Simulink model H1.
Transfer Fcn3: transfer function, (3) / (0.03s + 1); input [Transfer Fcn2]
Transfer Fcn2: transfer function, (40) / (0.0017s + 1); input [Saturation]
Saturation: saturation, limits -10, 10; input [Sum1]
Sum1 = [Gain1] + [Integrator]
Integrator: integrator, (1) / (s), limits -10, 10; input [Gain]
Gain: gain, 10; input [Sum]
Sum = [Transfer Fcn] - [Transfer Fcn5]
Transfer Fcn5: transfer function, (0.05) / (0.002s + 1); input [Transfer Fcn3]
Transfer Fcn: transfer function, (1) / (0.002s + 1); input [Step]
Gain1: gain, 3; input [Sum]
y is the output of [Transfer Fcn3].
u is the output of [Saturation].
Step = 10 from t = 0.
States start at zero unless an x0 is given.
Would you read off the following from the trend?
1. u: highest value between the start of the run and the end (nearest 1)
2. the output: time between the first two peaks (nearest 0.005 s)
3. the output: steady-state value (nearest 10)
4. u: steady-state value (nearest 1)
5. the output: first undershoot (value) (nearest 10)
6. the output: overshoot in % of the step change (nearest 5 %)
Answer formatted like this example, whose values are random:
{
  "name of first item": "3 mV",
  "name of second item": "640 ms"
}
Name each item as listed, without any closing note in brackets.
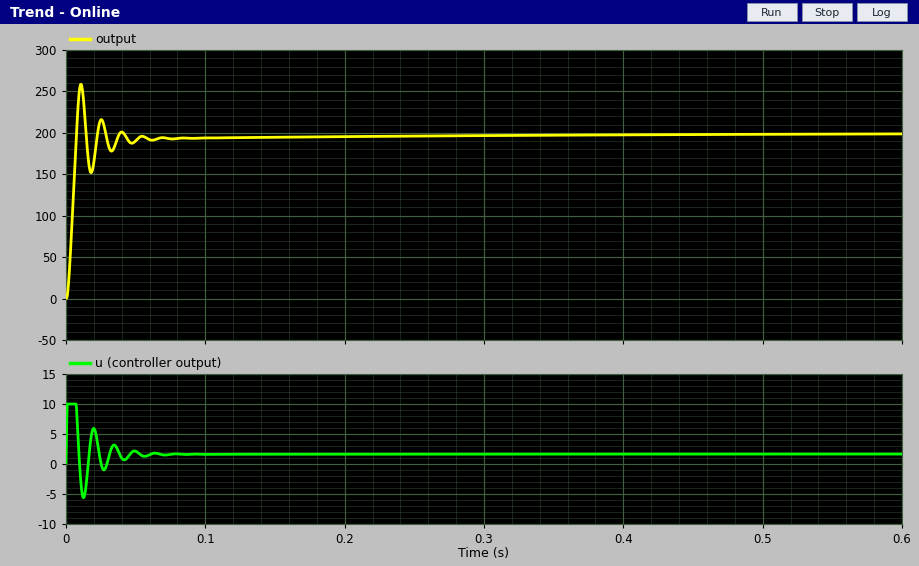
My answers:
{
  "u: highest value between the start of the run and the end": "10",
  "the output: time between the first two peaks": "0.015 s",
  "the output: steady-state value": "200",
  "u: steady-state value": "2",
  "the output: first undershoot (value)": "150",
  "the output: overshoot in % of the step change": "30 %"
}
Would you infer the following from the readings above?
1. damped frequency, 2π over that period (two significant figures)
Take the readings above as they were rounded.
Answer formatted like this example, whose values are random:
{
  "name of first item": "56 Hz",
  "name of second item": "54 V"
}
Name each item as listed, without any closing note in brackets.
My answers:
{
  "damped frequency, 2π over that period": "420 rad/s"
}
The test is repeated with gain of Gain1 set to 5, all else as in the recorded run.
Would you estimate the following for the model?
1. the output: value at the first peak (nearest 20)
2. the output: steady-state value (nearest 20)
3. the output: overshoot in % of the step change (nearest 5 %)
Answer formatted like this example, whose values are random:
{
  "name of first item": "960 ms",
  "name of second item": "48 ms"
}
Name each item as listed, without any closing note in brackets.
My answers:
{
  "the output: value at the first peak": "260",
  "the output: steady-state value": "200",
  "the output: overshoot in % of the step change": "35 %"
}
